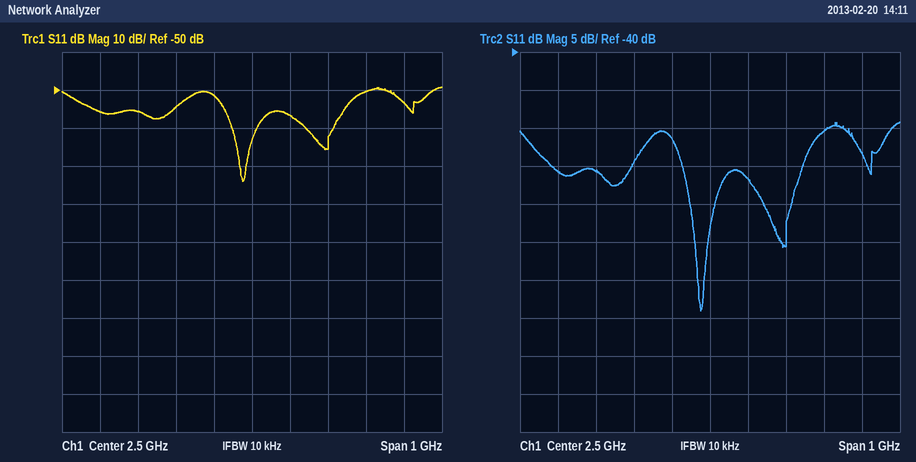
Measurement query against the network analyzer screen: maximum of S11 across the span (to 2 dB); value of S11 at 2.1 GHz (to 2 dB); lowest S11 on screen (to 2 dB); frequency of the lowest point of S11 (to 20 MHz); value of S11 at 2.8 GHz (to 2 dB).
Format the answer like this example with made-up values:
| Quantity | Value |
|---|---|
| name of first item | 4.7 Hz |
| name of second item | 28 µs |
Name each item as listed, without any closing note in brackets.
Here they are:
| Quantity | Value |
|---|---|
| maximum of S11 across the span | -50 dB |
| value of S11 at 2.1 GHz | -56 dB |
| lowest S11 on screen | -74 dB |
| frequency of the lowest point of S11 | 2.48 GHz |
| value of S11 at 2.8 GHz | -50 dB |
